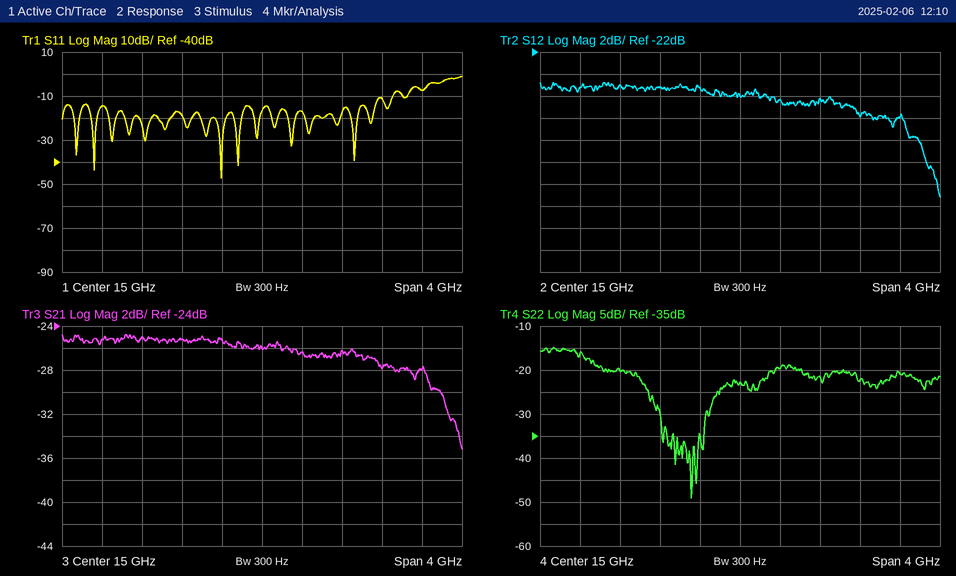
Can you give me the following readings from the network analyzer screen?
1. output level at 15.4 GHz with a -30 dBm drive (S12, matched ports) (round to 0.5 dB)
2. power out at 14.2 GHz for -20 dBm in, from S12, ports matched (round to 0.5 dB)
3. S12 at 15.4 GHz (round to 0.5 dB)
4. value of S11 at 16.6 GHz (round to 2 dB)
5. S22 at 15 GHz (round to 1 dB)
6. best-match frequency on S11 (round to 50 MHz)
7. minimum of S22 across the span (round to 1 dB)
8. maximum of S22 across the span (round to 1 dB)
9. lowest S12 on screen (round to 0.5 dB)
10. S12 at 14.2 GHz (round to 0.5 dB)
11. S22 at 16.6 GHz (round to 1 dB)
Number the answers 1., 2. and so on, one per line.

1. -56.5 dBm
2. -45.0 dBm
3. -26.5 dB
4. -8 dB
5. -23 dB
6. 14.60 GHz
7. -49 dB
8. -15 dB
9. -35.0 dB
10. -25.0 dB
11. -21 dB
